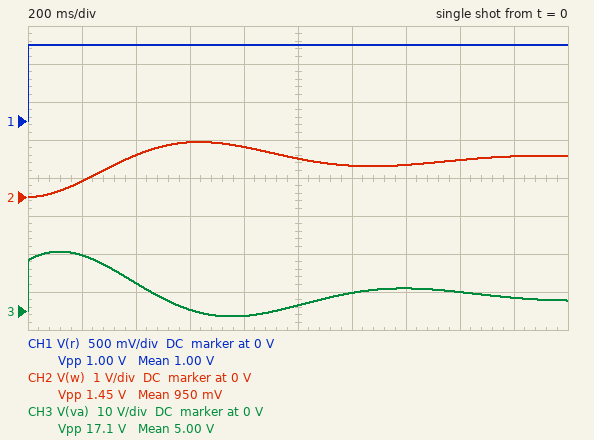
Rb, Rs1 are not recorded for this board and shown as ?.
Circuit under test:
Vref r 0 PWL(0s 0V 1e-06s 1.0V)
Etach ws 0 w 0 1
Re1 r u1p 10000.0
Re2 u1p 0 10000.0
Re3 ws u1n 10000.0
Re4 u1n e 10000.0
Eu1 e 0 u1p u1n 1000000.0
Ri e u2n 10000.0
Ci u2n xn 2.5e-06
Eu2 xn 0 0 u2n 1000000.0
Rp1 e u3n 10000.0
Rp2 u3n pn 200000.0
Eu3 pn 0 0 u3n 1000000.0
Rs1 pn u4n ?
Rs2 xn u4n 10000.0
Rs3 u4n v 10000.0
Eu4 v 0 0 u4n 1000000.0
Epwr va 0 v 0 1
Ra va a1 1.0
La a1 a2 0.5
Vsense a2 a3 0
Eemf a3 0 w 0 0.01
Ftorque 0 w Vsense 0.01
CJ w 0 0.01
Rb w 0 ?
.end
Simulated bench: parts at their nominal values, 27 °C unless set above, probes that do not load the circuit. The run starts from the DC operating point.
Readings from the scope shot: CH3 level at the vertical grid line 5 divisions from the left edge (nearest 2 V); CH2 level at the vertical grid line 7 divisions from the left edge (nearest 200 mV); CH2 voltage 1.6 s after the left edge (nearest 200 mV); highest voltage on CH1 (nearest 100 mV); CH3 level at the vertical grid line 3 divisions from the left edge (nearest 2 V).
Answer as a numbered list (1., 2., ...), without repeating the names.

1. 2 V
2. 800 mV
3. 1.0 V
4. 1.0 V
5. 0 V
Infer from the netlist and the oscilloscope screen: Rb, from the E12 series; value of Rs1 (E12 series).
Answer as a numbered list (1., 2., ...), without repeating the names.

1. 27 Ω
2. 15 kΩ
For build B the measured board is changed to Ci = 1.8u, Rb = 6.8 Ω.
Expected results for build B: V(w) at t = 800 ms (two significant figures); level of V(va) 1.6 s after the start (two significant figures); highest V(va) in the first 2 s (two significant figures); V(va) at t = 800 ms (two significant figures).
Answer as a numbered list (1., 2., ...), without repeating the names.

1. 1.0 V
2. 14 V
3. 21 V
4. 19 V
